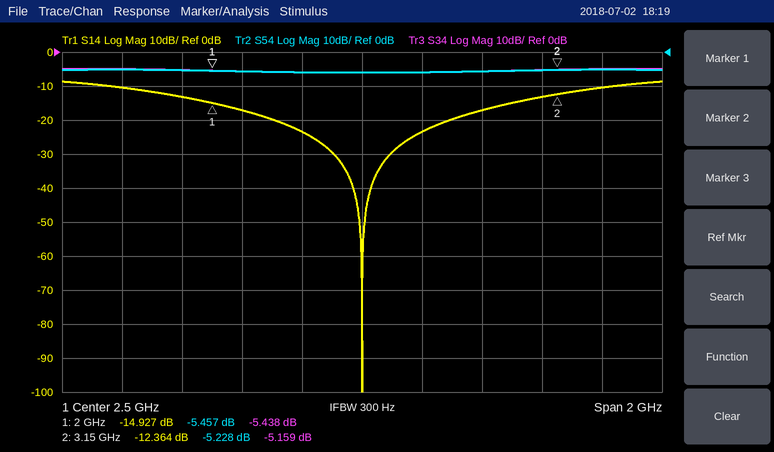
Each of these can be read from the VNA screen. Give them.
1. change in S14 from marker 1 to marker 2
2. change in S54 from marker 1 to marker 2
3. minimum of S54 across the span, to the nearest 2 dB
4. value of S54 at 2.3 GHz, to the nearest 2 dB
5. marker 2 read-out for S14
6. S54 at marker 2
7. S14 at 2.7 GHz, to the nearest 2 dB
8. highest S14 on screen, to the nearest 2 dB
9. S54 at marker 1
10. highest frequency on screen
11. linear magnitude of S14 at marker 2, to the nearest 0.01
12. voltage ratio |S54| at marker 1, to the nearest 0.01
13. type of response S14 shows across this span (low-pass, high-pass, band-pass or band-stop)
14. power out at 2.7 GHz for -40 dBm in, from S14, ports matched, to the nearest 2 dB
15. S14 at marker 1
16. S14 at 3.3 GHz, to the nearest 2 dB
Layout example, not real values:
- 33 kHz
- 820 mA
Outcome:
- 2.563 dB
- 0.229 dB
- -6 dB
- -6 dB
- -12.364 dB
- -5.228 dB
- -24 dB
- -8 dB
- -5.457 dB
- 3.5 GHz
- 0.24
- 0.53
- band-stop
- -64 dBm
- -14.927 dB
- -10 dB
